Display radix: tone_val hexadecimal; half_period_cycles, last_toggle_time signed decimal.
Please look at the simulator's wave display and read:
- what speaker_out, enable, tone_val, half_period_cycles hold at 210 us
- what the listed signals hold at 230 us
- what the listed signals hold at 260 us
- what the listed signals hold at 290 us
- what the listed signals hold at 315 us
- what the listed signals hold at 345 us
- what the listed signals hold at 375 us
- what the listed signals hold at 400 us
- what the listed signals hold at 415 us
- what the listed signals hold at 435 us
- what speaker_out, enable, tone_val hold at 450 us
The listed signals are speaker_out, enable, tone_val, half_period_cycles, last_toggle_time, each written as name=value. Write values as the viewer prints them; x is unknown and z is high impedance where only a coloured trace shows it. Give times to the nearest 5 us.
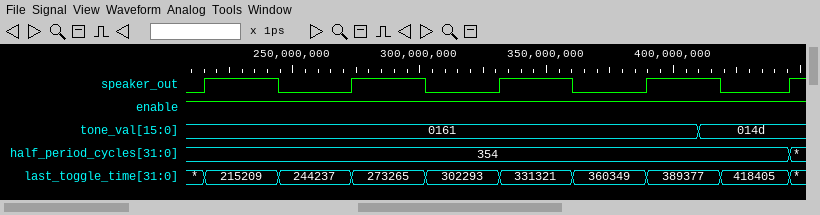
speaker_out=0, enable=1, tone_val=0161, half_period_cycles=354
speaker_out=1, enable=1, tone_val=0161, half_period_cycles=354, last_toggle_time=215209
speaker_out=0, enable=1, tone_val=0161, half_period_cycles=354, last_toggle_time=244237
speaker_out=1, enable=1, tone_val=0161, half_period_cycles=354, last_toggle_time=273265
speaker_out=0, enable=1, tone_val=0161, half_period_cycles=354, last_toggle_time=302293
speaker_out=1, enable=1, tone_val=0161, half_period_cycles=354, last_toggle_time=331321
speaker_out=0, enable=1, tone_val=0161, half_period_cycles=354, last_toggle_time=360349
speaker_out=1, enable=1, tone_val=0161, half_period_cycles=354, last_toggle_time=389377
speaker_out=1, enable=1, tone_val=014d, half_period_cycles=354, last_toggle_time=389377
speaker_out=0, enable=1, tone_val=014d, half_period_cycles=354, last_toggle_time=418405
speaker_out=1, enable=1, tone_val=014d
